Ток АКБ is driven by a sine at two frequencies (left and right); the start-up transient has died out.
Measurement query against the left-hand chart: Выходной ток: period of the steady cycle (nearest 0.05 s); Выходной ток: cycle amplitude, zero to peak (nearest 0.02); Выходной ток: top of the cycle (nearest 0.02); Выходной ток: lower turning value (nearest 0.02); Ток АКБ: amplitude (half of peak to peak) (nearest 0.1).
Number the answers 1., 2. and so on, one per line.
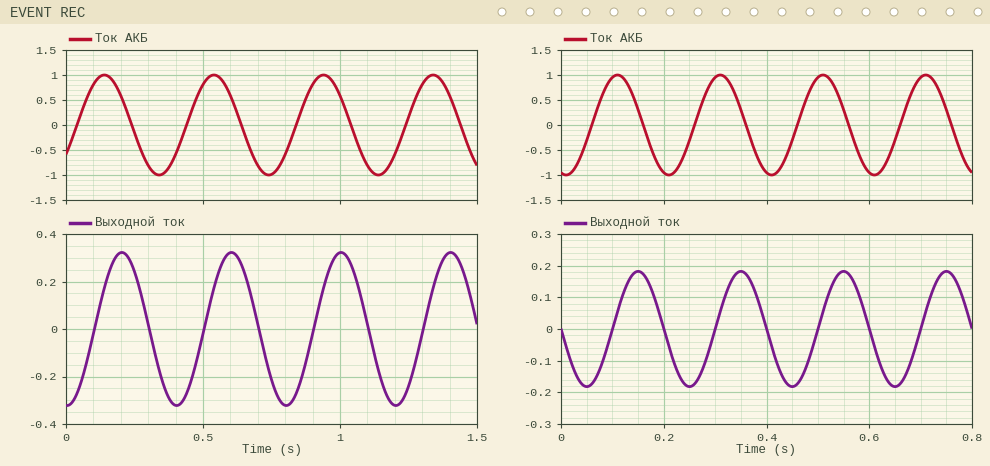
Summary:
1. 0.40 s
2. 0.32
3. 0.32
4. -0.32
5. 1.0
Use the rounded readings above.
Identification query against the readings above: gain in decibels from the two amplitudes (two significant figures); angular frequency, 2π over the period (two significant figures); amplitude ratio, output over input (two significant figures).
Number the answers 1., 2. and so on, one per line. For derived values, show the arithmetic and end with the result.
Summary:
1. 20 log10(0.32 / 1) = -9.9 dB
2. 2π / 0.4 = 16 rad/s
3. 0.32 / 1 = 0.32
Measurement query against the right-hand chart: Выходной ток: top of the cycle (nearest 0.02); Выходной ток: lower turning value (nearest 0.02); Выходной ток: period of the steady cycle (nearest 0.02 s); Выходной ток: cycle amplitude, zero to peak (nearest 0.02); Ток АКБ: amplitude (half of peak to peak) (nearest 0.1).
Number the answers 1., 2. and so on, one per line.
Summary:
1. 0.18
2. -0.18
3. 0.20 s
4. 0.18
5. 1.0
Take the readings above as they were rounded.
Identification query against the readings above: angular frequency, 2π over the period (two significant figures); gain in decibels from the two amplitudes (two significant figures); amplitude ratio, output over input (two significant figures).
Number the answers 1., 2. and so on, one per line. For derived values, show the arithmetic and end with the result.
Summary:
1. 2π / 0.2 = 31 rad/s
2. 20 log10(0.18 / 1) = -15 dB
3. 0.18 / 1 = 0.18
